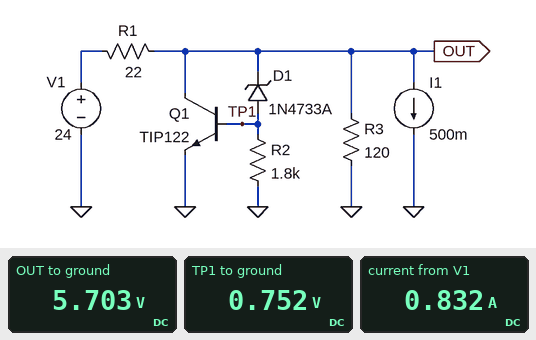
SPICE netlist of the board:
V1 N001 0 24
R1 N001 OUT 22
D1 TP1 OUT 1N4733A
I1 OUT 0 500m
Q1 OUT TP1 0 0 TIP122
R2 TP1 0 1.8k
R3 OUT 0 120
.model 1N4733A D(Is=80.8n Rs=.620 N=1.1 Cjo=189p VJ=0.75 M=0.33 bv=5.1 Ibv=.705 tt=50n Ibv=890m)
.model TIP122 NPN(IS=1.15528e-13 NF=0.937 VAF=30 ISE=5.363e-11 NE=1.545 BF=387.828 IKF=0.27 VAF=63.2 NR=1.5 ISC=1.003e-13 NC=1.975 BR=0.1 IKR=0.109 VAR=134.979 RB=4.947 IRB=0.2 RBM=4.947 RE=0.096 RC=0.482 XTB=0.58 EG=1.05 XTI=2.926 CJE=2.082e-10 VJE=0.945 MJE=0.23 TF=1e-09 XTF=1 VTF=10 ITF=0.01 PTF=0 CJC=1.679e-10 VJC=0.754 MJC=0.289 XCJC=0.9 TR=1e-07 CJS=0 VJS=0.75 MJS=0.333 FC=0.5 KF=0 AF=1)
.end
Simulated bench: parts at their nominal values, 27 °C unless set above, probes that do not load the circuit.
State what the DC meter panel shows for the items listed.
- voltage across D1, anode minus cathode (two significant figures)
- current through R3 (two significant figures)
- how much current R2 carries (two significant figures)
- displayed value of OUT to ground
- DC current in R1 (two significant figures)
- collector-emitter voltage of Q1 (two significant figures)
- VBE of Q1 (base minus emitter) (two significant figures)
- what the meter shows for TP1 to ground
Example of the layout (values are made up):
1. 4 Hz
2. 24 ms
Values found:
1. -5.0 V
2. 48 mA
3. 420 µA
4. 5.703 V
5. 830 mA
6. 5.7 V
7. 750 mV
8. 0.752 V
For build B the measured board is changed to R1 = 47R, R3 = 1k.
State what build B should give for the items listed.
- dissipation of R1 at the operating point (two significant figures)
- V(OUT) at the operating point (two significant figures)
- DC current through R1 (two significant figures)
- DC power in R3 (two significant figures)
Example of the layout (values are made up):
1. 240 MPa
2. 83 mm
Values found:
1. 12 W
2. 480 mV
3. 500 mA
4. 230 µW
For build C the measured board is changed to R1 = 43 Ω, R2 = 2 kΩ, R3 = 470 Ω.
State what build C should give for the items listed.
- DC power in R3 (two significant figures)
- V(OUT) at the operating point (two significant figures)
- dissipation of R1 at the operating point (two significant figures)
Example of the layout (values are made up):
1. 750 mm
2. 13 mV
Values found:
1. 11 mW
2. 2.3 V
3. 11 W
